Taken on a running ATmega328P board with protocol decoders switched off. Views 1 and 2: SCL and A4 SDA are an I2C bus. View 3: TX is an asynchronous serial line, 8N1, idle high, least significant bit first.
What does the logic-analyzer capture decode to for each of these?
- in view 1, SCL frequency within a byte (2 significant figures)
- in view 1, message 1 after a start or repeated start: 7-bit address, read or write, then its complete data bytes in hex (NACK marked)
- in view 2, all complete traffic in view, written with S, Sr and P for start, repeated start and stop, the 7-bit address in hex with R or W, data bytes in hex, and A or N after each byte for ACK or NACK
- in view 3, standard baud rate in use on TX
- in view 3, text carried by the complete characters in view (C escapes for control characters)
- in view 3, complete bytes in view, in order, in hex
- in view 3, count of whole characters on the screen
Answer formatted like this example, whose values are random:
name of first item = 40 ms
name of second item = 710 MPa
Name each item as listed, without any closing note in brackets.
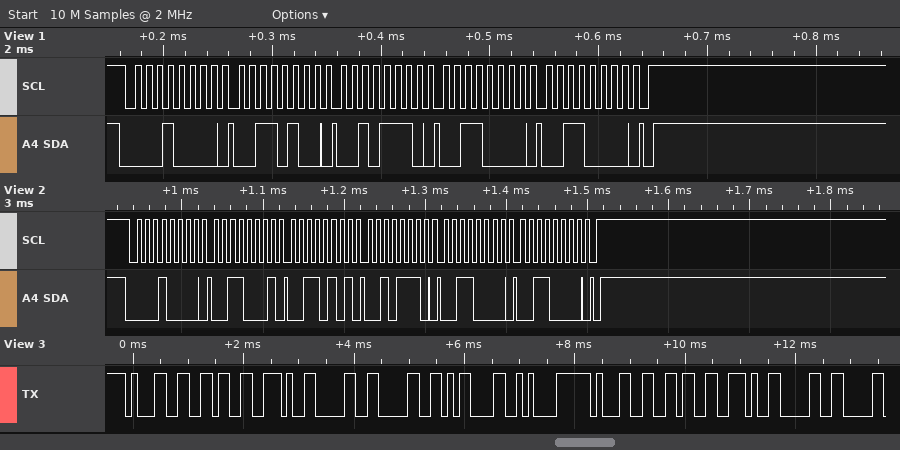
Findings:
in view 1, SCL frequency within a byte = 100 kHz
in view 1, message 1 after a start or repeated start: 7-bit address, read or write, then its complete data bytes in hex = 0x08 write: 34 2E 30 30
in view 2, all complete traffic in view, written with S, Sr and P for start, repeated start and stop, the 7-bit address in hex with R or W, data bytes in hex, and A or N after each byte for ACK or NACK = S 08W A 31 A 35 A 2E A 30 A 30 A P
in view 3, standard baud rate in use on TX = 9600 baud
in view 3, text carried by the complete characters in view = "16.00\r\n16.0"
in view 3, complete bytes in view, in order, in hex = 31 36 2E 30 30 0D 0A 31 36 2E 30
in view 3, count of whole characters on the screen = 11
